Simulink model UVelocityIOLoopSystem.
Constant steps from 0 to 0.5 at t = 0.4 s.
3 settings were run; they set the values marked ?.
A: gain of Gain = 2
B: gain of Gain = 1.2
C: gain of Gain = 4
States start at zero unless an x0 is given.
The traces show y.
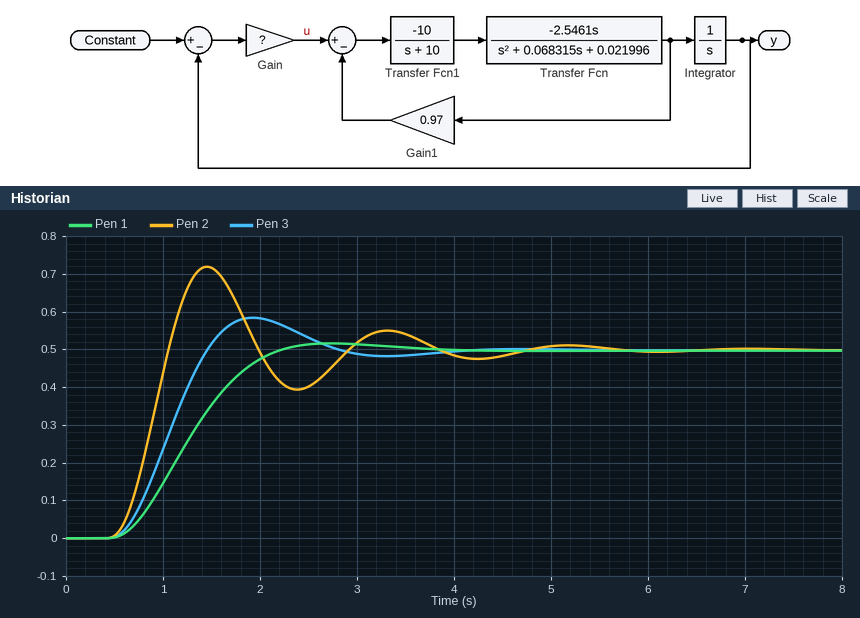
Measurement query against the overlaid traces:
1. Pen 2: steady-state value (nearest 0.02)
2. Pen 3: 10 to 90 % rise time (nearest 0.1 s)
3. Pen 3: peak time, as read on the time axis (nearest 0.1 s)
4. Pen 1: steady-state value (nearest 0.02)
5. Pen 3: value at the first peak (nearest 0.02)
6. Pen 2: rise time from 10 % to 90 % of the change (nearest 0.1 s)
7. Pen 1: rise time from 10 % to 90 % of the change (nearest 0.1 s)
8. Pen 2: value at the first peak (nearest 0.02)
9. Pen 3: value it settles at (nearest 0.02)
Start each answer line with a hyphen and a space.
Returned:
- 0.50
- 0.7 s
- 1.9 s
- 0.50
- 0.58
- 0.4 s
- 1.1 s
- 0.72
- 0.50
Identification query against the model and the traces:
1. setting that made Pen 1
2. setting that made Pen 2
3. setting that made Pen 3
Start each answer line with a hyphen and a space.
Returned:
- B
- C
- A
